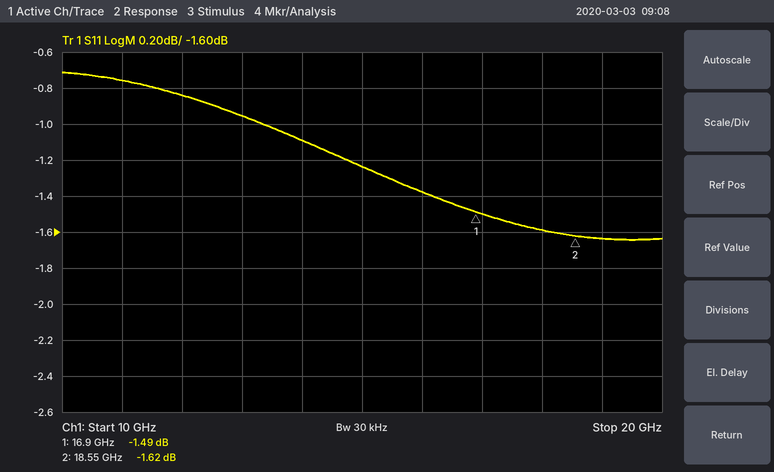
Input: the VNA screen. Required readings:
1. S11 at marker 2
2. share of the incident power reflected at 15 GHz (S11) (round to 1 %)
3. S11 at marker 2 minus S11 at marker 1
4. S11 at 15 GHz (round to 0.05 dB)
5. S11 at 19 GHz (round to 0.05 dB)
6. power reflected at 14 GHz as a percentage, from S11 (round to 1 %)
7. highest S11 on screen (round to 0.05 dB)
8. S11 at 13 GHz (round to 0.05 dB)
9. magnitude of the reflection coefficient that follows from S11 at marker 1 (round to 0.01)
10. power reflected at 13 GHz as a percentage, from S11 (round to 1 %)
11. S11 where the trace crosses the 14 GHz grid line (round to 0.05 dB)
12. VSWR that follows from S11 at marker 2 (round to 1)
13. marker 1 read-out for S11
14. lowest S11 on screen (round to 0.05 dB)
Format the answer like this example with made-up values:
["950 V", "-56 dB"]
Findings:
["-1.62 dB", "75 %", "-0.13 dB", "-1.25 dB", "-1.65 dB", "78 %", "-0.70 dB", "-0.95 dB", "0.84", "80 %", "-1.10 dB", "11", "-1.49 dB", "-1.65 dB"]
